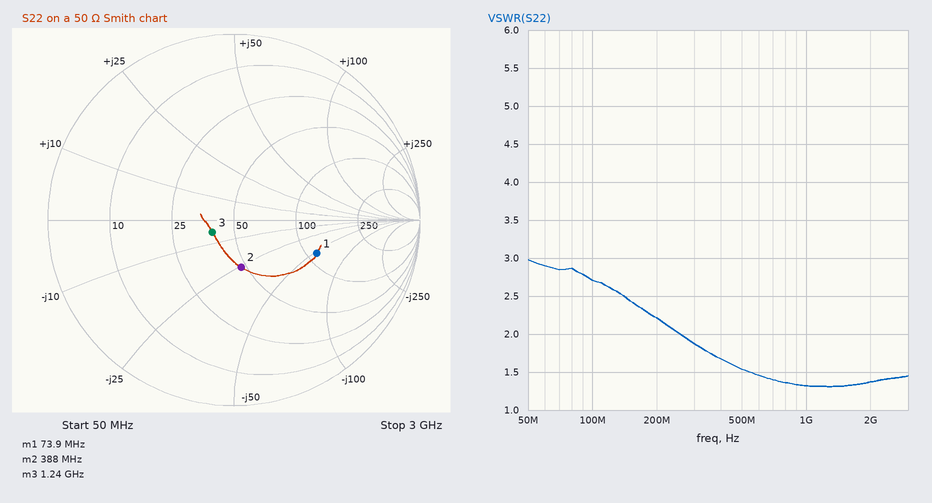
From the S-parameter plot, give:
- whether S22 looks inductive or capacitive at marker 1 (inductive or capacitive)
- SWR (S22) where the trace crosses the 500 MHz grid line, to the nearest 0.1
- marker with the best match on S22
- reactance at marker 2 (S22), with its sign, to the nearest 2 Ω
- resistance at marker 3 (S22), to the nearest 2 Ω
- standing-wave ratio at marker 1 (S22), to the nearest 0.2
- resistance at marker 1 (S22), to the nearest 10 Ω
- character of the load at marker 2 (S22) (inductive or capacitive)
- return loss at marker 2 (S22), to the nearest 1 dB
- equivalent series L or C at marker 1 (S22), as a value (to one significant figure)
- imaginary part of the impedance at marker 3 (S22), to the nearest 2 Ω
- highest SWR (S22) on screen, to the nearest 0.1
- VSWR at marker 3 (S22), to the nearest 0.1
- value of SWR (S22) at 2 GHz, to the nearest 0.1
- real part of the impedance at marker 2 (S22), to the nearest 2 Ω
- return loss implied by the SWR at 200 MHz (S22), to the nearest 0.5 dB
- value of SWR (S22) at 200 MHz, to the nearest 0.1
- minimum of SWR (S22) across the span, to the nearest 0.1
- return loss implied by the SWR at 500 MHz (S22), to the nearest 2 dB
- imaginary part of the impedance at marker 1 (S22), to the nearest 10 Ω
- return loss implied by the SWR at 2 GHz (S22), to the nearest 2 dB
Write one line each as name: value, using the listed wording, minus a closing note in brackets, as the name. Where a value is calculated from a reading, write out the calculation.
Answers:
whether S22 looks inductive or capacitive at marker 1: capacitive
SWR (S22) where the trace crosses the 500 MHz grid line, to the nearest 0.1: 1.5
marker with the best match on S22: marker 3
reactance at marker 2 (S22), with its sign, to the nearest 2 Ω: -26 Ω
resistance at marker 3 (S22), to the nearest 2 Ω: 40 Ω
standing-wave ratio at marker 1 (S22), to the nearest 0.2: 2.8
resistance at marker 1 (S22), to the nearest 10 Ω: 110 Ω
character of the load at marker 2 (S22): capacitive
return loss at marker 2 (S22), to the nearest 1 dB: 12 dB
equivalent series L or C at marker 1 (S22), as a value: C = 1/(2π × 73.9 MHz × 50 Ω) ≈ 43.1 pF, so 40 pF to one significant figure
imaginary part of the impedance at marker 3 (S22), to the nearest 2 Ω: -6 Ω
highest SWR (S22) on screen, to the nearest 0.1: 3.0
VSWR at marker 3 (S22), to the nearest 0.1: 1.3
value of SWR (S22) at 2 GHz, to the nearest 0.1: 1.4
real part of the impedance at marker 2 (S22), to the nearest 2 Ω: 48 Ω
return loss implied by the SWR at 200 MHz (S22), to the nearest 0.5 dB: −20 log10((2.2 − 1)/(2.2 + 1)) ≈ 8.5 dB
value of SWR (S22) at 200 MHz, to the nearest 0.1: 2.2
minimum of SWR (S22) across the span, to the nearest 0.1: 1.3
return loss implied by the SWR at 500 MHz (S22), to the nearest 2 dB: −20 log10((1.5 − 1)/(1.5 + 1)) ≈ 14 dB
imaginary part of the impedance at marker 1 (S22), to the nearest 10 Ω: -50 Ω
return loss implied by the SWR at 2 GHz (S22), to the nearest 2 dB: −20 log10((1.4 − 1)/(1.4 + 1)) ≈ 16 dB
